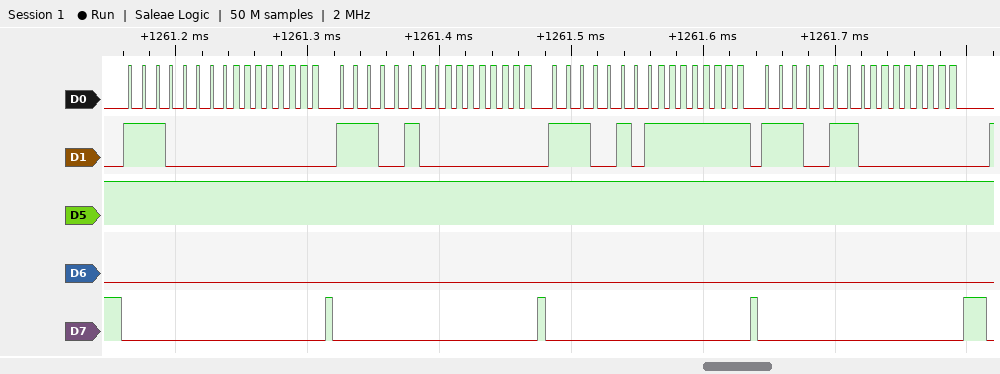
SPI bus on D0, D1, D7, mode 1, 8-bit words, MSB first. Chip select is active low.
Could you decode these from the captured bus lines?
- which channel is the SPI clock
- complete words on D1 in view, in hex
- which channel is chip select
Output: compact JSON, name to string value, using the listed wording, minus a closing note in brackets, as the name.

{"which channel is the SPI clock": "D0", "complete words on D1 in view, in hex": "E0, 00, E4, 00, E5, FF, E6, 00", "which channel is chip select": "D7"}
